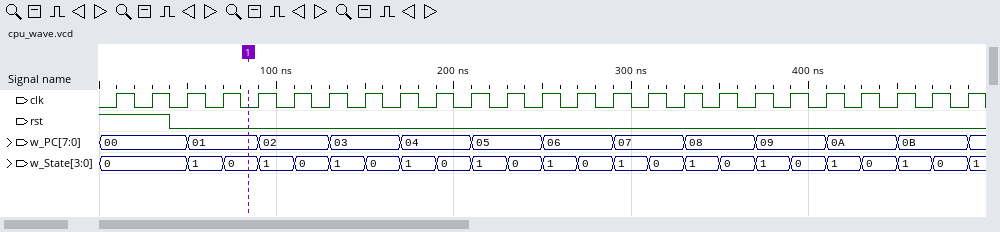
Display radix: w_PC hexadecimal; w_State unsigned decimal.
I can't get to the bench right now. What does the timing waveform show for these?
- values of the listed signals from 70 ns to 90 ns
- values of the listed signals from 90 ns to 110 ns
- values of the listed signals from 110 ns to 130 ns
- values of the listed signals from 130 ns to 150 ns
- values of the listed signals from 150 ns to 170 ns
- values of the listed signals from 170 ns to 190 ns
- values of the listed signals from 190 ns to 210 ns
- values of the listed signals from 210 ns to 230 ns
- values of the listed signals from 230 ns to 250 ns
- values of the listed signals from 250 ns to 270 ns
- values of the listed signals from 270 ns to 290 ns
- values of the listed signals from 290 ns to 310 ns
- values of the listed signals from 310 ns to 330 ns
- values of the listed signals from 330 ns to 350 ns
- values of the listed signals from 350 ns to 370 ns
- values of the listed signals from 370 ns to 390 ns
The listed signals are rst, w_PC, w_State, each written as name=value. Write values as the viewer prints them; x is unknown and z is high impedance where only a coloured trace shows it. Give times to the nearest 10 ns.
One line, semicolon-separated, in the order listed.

rst=0, w_PC=01, w_State=0; rst=0, w_PC=02, w_State=1; rst=0, w_PC=02, w_State=0; rst=0, w_PC=03, w_State=1; rst=0, w_PC=03, w_State=0; rst=0, w_PC=04, w_State=1; rst=0, w_PC=04, w_State=0; rst=0, w_PC=05, w_State=1; rst=0, w_PC=05, w_State=0; rst=0, w_PC=06, w_State=1; rst=0, w_PC=06, w_State=0; rst=0, w_PC=07, w_State=1; rst=0, w_PC=07, w_State=0; rst=0, w_PC=08, w_State=1; rst=0, w_PC=08, w_State=0; rst=0, w_PC=09, w_State=1
